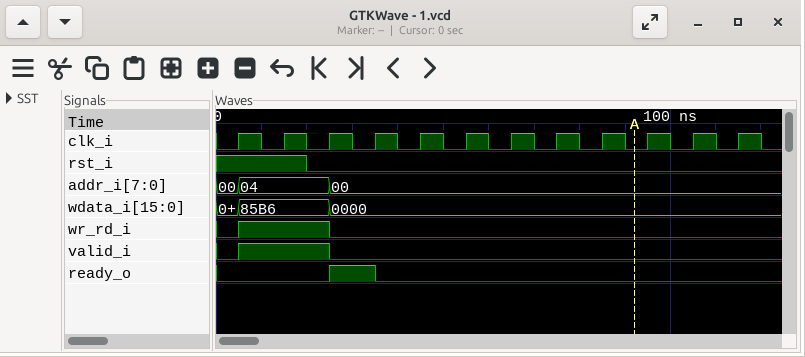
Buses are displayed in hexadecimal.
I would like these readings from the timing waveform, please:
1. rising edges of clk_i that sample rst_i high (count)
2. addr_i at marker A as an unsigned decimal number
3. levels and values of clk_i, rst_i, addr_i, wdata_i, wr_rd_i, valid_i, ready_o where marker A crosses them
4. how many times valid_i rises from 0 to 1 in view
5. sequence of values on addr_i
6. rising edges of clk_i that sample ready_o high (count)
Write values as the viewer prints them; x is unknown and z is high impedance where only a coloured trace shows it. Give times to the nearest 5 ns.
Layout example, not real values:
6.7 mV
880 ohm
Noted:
2
0
clk_i=0, rst_i=0, addr_i=00, wdata_i=0000, wr_rd_i=0, valid_i=0, ready_o=0
1
00, 04, 00
1
